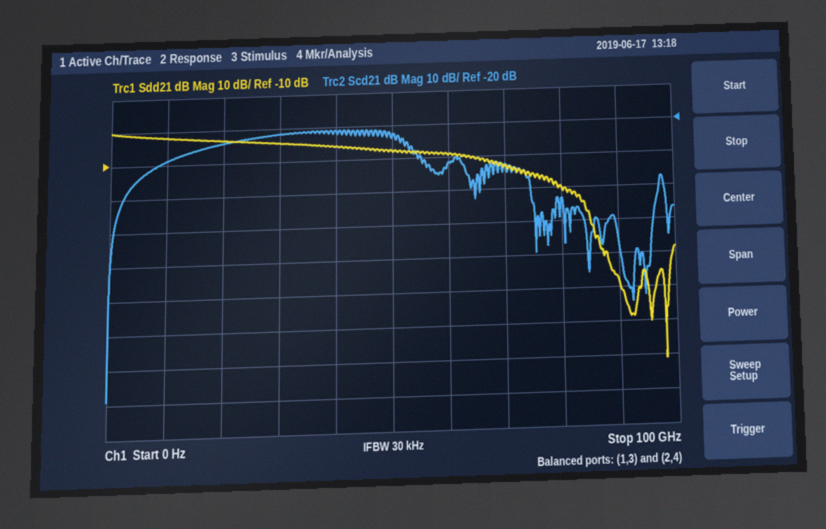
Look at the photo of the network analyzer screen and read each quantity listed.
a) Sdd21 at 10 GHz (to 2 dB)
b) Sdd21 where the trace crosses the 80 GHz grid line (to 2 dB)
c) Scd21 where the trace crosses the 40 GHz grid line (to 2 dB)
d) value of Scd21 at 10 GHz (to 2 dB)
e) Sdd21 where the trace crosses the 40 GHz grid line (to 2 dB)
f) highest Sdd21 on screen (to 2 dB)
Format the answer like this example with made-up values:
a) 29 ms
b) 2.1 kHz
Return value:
a) -2 dB
b) -20 dB
c) -22 dB
d) -28 dB
e) -6 dB
f) 0 dB
